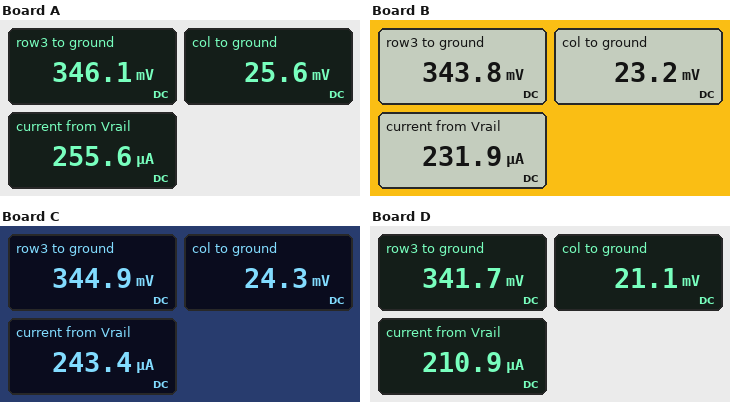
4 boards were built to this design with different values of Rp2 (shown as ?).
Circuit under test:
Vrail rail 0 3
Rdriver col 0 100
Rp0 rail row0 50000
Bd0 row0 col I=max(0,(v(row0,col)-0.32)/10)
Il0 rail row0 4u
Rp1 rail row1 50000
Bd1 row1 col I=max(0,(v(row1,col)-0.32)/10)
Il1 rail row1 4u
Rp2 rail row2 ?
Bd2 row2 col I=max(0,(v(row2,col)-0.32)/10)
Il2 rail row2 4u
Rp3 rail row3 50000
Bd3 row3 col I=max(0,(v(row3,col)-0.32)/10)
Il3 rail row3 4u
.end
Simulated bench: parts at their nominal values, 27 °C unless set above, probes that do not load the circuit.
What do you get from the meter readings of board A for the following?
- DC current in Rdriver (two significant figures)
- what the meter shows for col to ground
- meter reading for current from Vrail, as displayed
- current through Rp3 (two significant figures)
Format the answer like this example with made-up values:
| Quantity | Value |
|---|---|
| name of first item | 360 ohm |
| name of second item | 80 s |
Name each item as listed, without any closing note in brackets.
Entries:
| Quantity | Value |
|---|---|
| DC current in Rdriver | 260 µA |
| what the meter shows for col to ground | 25.6 mV |
| meter reading for current from Vrail, as displayed | 255.6 µA |
| current through Rp3 | 53 µA |
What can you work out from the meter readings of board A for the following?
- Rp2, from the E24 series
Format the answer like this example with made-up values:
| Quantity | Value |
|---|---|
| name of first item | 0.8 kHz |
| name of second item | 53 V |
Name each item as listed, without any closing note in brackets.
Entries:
| Quantity | Value |
|---|---|
| Rp2, from the E24 series | 33 kΩ |
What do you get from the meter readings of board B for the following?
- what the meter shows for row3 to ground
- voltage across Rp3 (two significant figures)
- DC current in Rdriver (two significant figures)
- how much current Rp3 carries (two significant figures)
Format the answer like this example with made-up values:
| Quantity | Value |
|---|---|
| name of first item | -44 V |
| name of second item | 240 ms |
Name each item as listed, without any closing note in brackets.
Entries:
| Quantity | Value |
|---|---|
| what the meter shows for row3 to ground | 343.8 mV |
| voltage across Rp3 | 2.7 V |
| DC current in Rdriver | 230 µA |
| how much current Rp3 carries | 53 µA |
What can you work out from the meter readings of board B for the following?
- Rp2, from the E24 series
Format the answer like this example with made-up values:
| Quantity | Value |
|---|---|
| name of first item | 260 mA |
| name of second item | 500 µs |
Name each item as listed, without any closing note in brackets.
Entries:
| Quantity | Value |
|---|---|
| Rp2, from the E24 series | 47 kΩ |
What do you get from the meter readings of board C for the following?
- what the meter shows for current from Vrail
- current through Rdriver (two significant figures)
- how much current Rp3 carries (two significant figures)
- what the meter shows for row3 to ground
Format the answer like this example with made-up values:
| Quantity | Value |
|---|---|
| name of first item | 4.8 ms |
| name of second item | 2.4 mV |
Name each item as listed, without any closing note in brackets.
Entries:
| Quantity | Value |
|---|---|
| what the meter shows for current from Vrail | 243.4 µA |
| current through Rdriver | 240 µA |
| how much current Rp3 carries | 53 µA |
| what the meter shows for row3 to ground | 344.9 mV |
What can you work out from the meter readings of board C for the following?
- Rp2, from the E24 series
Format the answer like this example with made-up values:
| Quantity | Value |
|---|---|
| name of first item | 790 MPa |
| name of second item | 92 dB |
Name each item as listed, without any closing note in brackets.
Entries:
| Quantity | Value |
|---|---|
| Rp2, from the E24 series | 39 kΩ |
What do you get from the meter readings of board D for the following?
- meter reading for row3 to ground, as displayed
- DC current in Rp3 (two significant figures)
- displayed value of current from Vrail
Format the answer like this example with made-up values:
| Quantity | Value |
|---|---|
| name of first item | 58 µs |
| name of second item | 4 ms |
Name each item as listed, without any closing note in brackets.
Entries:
| Quantity | Value |
|---|---|
| meter reading for row3 to ground, as displayed | 341.7 mV |
| DC current in Rp3 | 53 µA |
| displayed value of current from Vrail | 210.9 µA |
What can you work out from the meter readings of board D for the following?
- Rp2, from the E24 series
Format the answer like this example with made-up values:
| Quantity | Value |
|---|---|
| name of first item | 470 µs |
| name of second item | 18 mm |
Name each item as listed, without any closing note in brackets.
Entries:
| Quantity | Value |
|---|---|
| Rp2, from the E24 series | 75 kΩ |
